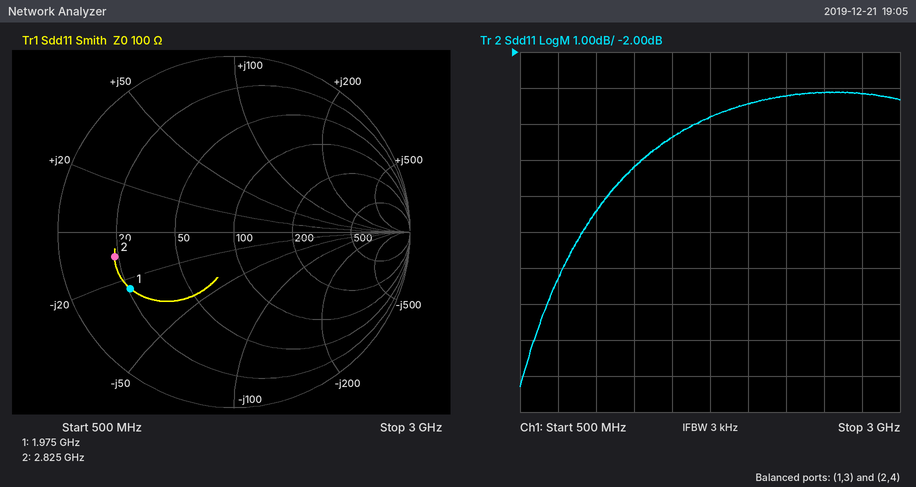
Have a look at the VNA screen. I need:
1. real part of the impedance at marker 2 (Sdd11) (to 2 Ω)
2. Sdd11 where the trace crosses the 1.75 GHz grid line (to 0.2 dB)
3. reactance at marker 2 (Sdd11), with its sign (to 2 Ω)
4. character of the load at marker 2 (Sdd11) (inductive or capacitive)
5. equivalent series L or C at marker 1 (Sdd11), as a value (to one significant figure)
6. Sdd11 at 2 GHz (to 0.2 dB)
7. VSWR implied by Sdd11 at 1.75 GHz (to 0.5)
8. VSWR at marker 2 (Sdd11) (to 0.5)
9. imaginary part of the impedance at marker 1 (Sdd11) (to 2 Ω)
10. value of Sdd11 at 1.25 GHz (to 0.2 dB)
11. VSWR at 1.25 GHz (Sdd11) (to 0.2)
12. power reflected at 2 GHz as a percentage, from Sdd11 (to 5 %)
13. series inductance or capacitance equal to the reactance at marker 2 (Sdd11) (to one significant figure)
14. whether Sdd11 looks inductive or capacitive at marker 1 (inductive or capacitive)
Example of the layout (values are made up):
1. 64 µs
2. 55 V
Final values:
1. 18 Ω
2. -3.8 dB
3. -10 Ω
4. capacitive
5. 3 pF
6. -3.4 dB
7. 4.5
8. 5.5
9. -24 Ω
10. -5.2 dB
11. 3.4
12. 45 %
13. 6 pF
14. capacitive
